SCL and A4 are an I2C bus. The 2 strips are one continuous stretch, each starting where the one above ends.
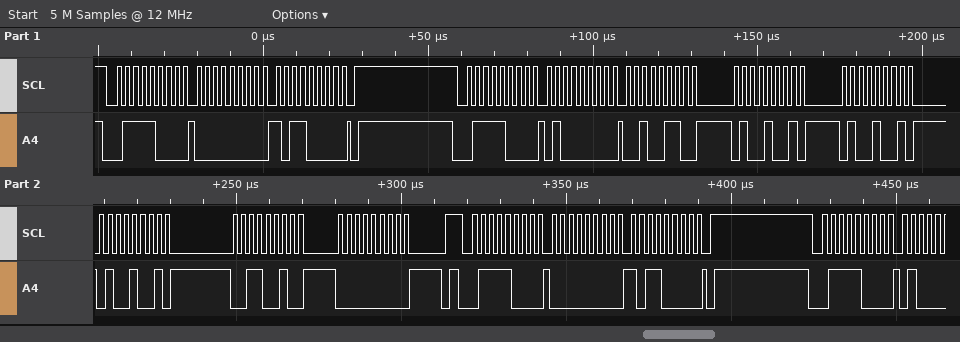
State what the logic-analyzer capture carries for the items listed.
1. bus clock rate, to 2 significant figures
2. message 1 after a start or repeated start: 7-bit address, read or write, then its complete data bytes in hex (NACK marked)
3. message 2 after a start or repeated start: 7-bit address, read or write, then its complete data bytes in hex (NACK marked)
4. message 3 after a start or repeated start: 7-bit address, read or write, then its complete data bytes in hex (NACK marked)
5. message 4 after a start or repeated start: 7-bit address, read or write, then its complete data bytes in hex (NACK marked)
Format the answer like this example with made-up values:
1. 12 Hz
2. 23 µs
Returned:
1. 400 kHz
2. 0x3C write: 00 B0
3. 0x3C write: 40 26 49 49 49 32 00
4. 0x3C write: 00 B0
5. 0x3C write
